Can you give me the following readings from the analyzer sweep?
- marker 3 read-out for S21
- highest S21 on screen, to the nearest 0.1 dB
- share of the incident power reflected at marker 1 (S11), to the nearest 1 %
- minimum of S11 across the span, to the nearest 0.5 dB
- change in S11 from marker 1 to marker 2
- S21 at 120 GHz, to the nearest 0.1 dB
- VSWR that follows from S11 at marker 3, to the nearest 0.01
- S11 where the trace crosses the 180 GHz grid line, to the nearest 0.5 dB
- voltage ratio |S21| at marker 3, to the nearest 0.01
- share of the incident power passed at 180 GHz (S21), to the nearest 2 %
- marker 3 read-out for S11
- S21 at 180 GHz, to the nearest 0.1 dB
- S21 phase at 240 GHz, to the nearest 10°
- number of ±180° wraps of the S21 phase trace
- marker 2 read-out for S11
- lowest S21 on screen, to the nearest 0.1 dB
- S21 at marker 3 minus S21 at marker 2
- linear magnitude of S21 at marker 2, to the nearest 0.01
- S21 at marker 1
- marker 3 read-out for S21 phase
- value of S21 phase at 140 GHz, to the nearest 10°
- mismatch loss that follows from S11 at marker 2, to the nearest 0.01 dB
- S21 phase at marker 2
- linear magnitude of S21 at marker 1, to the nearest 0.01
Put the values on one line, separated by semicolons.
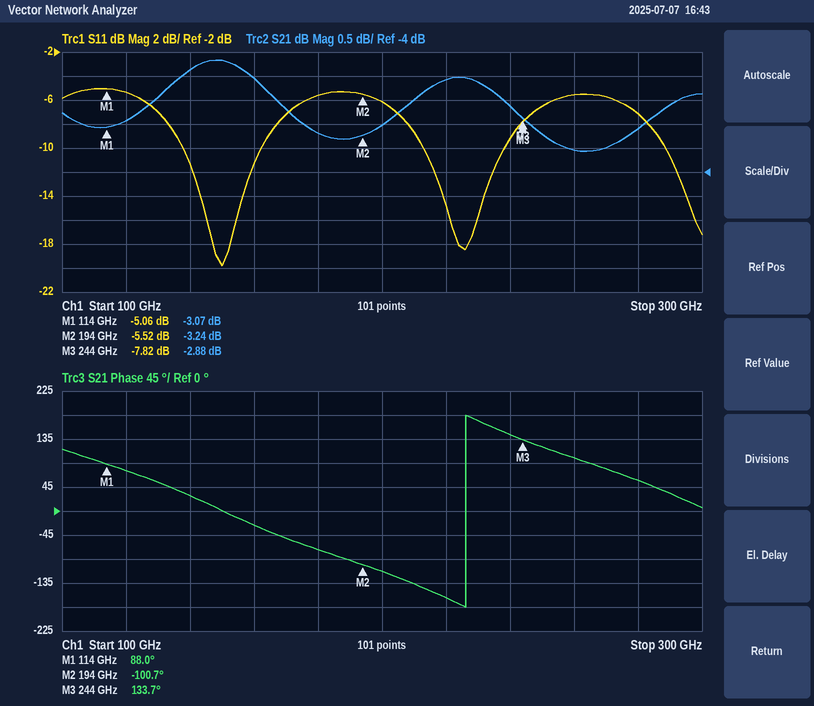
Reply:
-2.88 dB; -1.7 dB; 31 %; -20.0 dB; -0.46 dB; -2.9 dB; 2.37; -5.5 dB; 0.72; 48 %; -7.82 dB; -3.2 dB; 140°; 1; -5.52 dB; -3.6 dB; 0.36 dB; 0.69; -3.07 dB; 133.7°; 30°; 1.43 dB; -100.7°; 0.70
